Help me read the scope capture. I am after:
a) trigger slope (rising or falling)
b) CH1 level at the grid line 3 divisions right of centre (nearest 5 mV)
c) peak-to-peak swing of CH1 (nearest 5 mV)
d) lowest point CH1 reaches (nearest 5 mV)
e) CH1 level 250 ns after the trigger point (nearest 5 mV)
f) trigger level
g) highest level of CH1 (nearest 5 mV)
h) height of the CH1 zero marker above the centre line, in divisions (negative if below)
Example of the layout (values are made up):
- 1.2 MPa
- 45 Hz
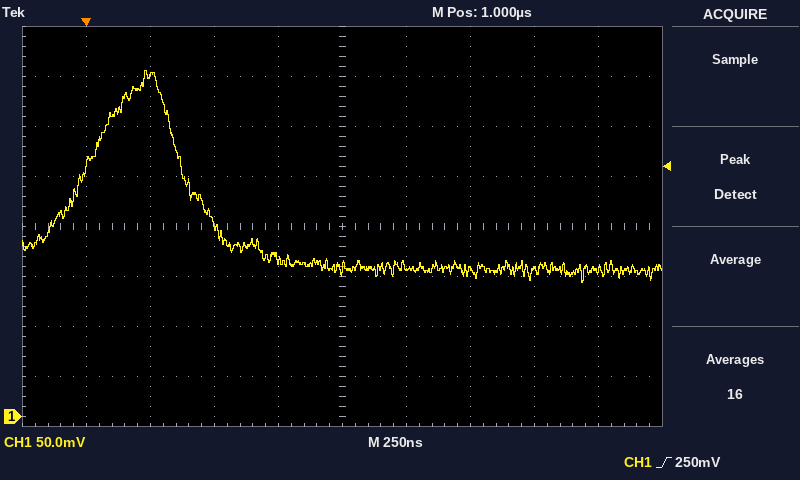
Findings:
- rising
- 145 mV
- 210 mV
- 135 mV
- 340 mV
- 250 mV
- 345 mV
- -3.8 div
